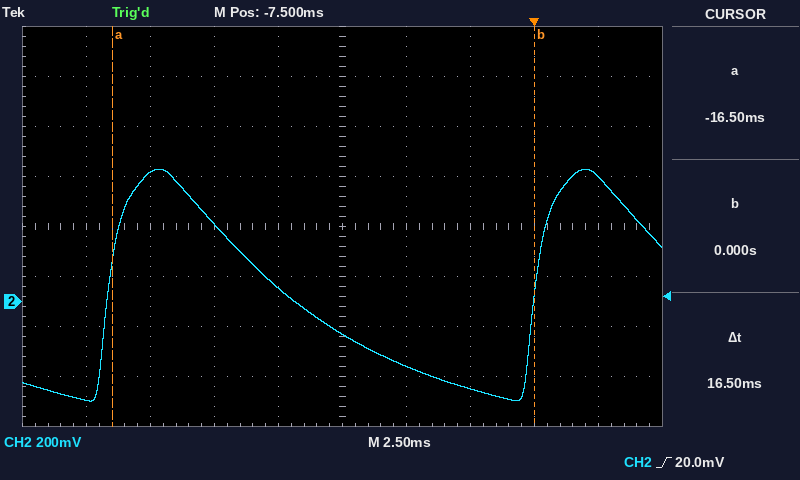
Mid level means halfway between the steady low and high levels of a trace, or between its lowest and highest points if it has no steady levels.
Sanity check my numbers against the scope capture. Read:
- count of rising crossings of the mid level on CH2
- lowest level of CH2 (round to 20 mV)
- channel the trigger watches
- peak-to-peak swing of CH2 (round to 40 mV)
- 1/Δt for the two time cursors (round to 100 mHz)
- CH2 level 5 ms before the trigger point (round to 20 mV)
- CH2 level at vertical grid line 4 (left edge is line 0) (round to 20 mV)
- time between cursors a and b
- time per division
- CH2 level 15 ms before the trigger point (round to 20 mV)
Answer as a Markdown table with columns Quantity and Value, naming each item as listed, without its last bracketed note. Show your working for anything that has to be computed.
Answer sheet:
| Quantity | Value |
|---|---|
| count of rising crossings of the mid level on CH2 | 2 |
| lowest level of CH2 | -400 mV |
| channel the trigger watches | CH2 |
| peak-to-peak swing of CH2 | 920 mV |
| 1/Δt for the two time cursors | 1 / 16.5 ms ≈ 60.6 Hz |
| CH2 level 5 ms before the trigger point | -260 mV |
| CH2 level at vertical grid line 4 (left edge is line 0) | 60 mV |
| time between cursors a and b | 16.5 ms |
| time per division | 2.5 ms |
| CH2 level 15 ms before the trigger point | 520 mV |
